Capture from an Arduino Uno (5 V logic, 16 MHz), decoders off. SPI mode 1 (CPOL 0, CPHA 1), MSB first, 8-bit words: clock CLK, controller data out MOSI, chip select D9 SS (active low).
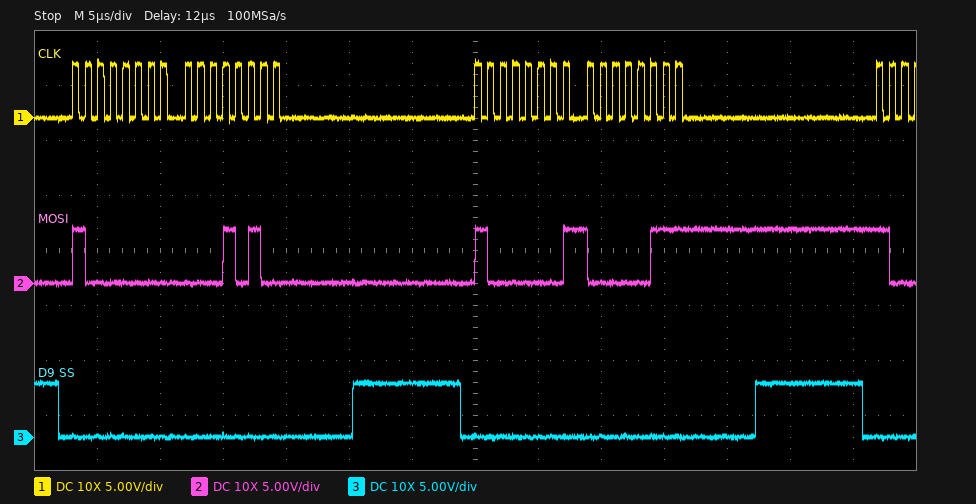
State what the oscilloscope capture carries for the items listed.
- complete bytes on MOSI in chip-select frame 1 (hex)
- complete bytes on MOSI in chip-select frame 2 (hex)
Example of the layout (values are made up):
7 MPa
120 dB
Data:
80 14
81 07
